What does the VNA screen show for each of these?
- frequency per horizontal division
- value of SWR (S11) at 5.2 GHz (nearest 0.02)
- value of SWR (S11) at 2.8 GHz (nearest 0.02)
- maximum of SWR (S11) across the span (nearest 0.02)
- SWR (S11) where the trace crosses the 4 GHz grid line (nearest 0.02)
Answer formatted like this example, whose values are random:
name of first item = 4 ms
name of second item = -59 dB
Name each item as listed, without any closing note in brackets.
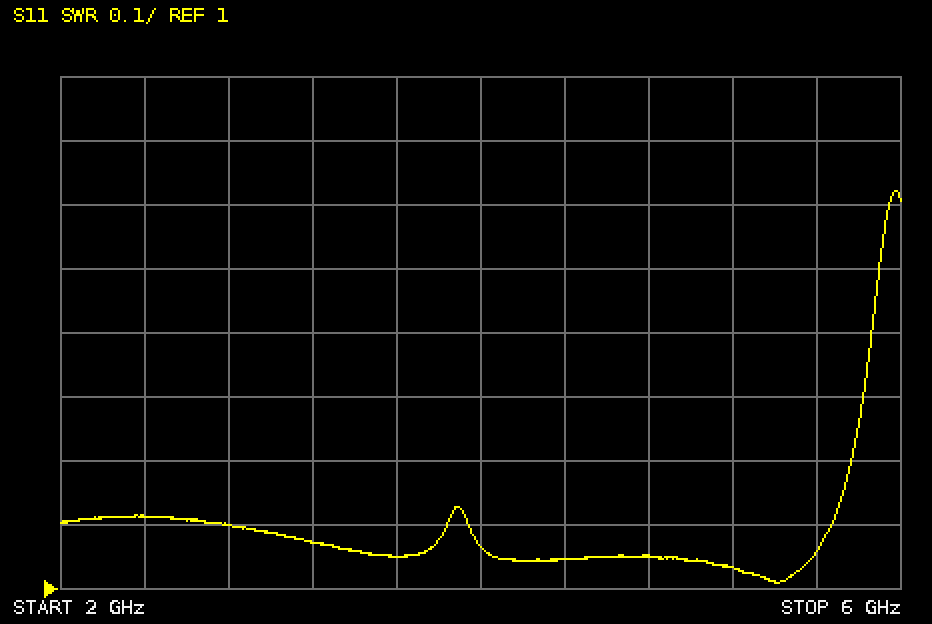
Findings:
frequency per horizontal division = 400 MHz
value of SWR (S11) at 5.2 GHz = 1.04
value of SWR (S11) at 2.8 GHz = 1.10
maximum of SWR (S11) across the span = 1.62
SWR (S11) where the trace crosses the 4 GHz grid line = 1.06
